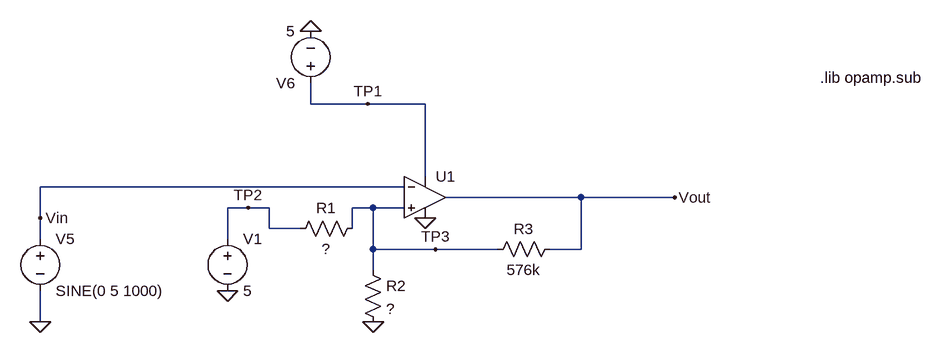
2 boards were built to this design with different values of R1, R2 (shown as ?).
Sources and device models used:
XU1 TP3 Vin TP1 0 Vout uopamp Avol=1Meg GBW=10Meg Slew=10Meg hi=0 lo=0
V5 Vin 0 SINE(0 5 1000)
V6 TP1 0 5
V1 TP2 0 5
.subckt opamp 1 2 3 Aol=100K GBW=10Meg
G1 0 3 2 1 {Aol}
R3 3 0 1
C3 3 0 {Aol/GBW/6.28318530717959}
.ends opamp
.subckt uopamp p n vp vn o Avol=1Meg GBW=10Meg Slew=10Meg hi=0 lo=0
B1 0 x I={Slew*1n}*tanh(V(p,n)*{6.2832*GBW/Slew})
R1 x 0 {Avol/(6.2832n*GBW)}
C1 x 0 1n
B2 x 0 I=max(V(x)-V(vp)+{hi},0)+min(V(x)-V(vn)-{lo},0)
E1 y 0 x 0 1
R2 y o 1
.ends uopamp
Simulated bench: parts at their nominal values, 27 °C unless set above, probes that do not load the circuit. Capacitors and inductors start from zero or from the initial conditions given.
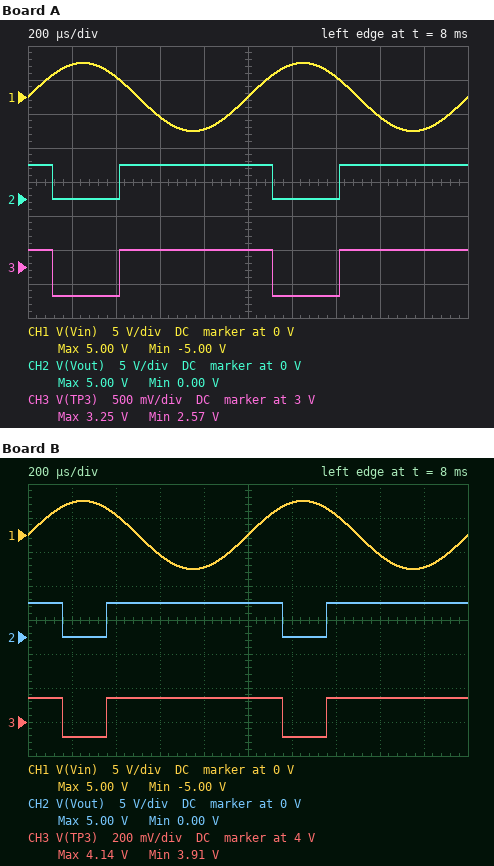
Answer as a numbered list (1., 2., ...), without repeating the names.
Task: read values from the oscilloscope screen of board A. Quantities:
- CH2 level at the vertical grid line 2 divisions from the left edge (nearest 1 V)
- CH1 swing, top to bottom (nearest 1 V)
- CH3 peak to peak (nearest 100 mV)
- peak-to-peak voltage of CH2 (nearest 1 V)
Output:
1. 0 V
2. 10 V
3. 700 mV
4. 5 V
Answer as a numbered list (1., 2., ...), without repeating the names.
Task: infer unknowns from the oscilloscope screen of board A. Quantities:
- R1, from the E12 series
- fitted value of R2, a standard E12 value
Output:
1. 150 kΩ
2. 220 kΩ
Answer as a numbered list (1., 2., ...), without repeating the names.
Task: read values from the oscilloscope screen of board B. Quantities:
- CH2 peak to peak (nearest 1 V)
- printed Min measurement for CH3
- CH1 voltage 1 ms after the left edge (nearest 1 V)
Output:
1. 5 V
2. 3.91 V
3. 0 V
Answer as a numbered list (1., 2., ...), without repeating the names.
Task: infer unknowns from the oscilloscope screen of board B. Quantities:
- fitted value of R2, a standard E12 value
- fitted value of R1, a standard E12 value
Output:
1. 150 kΩ
2. 33 kΩ
